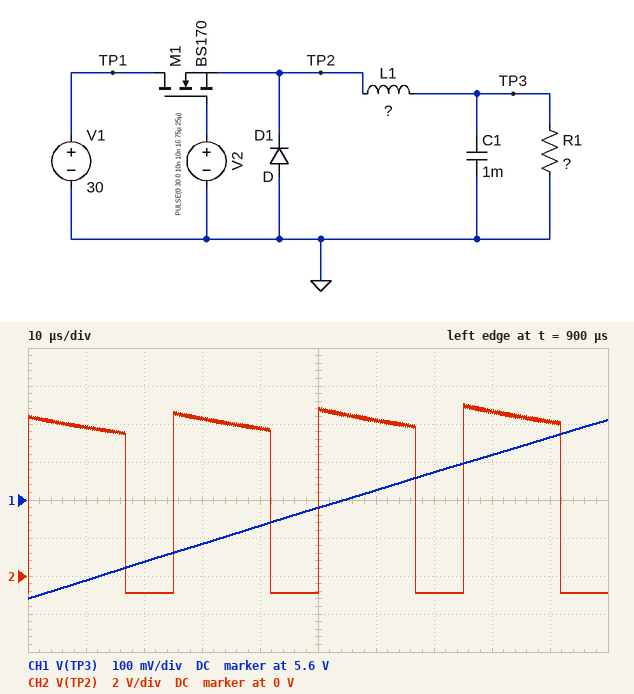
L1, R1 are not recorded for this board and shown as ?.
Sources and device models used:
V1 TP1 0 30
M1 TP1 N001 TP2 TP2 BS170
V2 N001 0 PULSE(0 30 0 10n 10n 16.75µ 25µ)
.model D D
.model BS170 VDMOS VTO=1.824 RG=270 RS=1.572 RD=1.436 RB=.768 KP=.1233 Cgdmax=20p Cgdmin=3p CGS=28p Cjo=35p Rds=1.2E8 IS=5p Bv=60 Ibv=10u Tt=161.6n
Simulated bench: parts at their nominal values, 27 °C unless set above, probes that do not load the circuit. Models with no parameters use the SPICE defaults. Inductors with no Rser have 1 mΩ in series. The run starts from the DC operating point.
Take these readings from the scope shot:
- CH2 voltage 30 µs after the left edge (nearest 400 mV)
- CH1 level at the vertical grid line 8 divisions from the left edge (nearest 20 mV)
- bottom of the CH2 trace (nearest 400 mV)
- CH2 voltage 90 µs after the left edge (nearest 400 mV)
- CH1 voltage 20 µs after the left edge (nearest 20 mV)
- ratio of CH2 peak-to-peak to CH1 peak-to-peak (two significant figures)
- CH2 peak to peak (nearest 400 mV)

8.4 V
5.72 V
-800 mV
8.0 V
5.44 V
21
10.0 V
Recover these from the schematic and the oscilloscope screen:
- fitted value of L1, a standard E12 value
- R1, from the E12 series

150 µH
6.8 Ω
